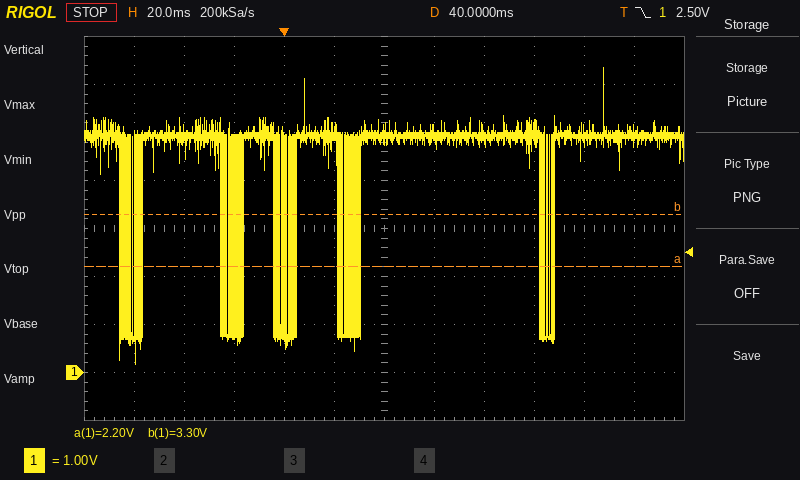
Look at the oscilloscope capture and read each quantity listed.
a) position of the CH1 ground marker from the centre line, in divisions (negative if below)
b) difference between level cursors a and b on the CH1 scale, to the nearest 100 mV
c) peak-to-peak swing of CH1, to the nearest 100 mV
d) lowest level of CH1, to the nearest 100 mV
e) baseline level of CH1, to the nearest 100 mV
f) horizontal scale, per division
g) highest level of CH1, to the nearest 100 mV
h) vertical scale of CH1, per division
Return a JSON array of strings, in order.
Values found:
["-3.0 div", "1.1 V", "6.2 V", "200 mV", "4.9 V", "20 ms", "6.4 V", "1 V"]
